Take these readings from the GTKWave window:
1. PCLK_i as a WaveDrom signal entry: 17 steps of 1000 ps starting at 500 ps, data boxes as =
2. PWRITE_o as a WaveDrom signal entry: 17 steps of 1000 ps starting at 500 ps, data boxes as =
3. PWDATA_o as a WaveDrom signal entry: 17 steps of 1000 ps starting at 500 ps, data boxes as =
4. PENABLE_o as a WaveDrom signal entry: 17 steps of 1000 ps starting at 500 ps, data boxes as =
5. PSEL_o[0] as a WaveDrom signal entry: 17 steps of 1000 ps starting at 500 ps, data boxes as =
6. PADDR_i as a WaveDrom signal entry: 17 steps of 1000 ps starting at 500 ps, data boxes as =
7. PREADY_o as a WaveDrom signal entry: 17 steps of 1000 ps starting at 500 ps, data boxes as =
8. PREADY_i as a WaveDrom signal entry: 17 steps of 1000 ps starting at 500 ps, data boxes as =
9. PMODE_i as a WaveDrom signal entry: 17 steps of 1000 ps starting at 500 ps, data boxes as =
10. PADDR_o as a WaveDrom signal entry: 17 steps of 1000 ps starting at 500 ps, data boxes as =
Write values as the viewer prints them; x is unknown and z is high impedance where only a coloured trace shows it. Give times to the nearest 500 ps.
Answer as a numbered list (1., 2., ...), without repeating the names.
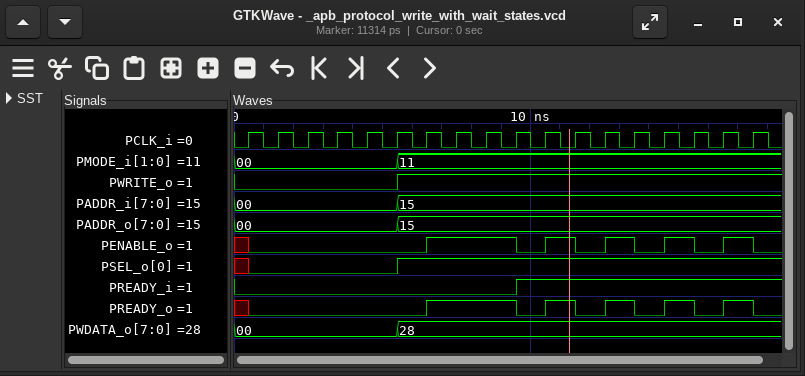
1. {name: 'PCLK_i', wave: 'p................'}
2. {name: 'PWRITE_o', wave: '0....1...........'}
3. {name: 'PWDATA_o', wave: '=....=...........', data: '00 28'}
4. {name: 'PENABLE_o', wave: '0.....1..01010101'}
5. {name: 'PSEL_o[0]', wave: '0....1...........'}
6. {name: 'PADDR_i', wave: '=....=...........', data: '00 15'}
7. {name: 'PREADY_o', wave: '0.....1..01010101'}
8. {name: 'PREADY_i', wave: '0........1.......'}
9. {name: 'PMODE_i', wave: '=....=...........', data: '00 11'}
10. {name: 'PADDR_o', wave: '=....=...........', data: '00 15'}
